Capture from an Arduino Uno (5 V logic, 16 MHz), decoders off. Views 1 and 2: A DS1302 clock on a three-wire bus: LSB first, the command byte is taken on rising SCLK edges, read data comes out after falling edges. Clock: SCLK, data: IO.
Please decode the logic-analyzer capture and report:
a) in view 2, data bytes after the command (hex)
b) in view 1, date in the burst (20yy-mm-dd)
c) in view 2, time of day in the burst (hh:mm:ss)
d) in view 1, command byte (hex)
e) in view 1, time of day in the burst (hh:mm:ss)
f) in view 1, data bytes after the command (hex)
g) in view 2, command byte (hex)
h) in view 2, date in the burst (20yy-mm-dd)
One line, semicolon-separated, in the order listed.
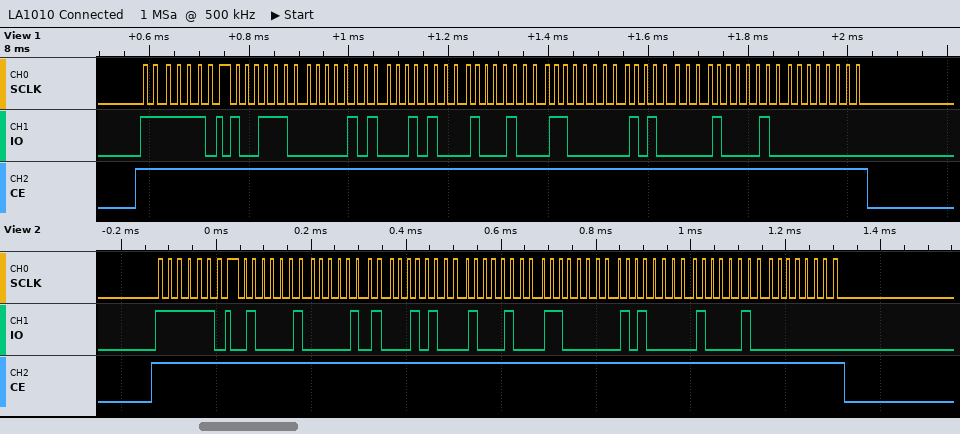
42 50 14 11 03 05 21 00; 2021-03-11; 14:50:42; 0xBF; 14:50:39; 39 50 14 11 03 05 21 00; 0xBF; 2021-03-11
